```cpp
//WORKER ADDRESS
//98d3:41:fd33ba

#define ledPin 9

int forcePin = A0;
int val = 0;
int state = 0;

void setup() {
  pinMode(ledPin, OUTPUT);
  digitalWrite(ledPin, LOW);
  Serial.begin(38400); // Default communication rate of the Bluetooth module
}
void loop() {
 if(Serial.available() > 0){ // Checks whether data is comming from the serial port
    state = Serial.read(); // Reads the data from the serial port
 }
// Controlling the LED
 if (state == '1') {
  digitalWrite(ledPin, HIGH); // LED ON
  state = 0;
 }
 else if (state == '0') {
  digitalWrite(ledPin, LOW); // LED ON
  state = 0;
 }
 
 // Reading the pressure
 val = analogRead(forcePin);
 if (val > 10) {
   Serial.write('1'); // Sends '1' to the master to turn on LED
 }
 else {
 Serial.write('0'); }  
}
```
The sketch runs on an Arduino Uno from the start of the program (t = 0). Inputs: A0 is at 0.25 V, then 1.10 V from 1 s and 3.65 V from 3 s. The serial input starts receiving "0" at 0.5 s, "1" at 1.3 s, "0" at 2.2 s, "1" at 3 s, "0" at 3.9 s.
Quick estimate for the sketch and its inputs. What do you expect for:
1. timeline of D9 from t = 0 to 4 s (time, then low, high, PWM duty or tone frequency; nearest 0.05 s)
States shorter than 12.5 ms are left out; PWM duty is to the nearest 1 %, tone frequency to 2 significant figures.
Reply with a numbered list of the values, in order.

1. 0 s low; 1.3 s high; 2.2 s low; 3 s high; 3.9 s low
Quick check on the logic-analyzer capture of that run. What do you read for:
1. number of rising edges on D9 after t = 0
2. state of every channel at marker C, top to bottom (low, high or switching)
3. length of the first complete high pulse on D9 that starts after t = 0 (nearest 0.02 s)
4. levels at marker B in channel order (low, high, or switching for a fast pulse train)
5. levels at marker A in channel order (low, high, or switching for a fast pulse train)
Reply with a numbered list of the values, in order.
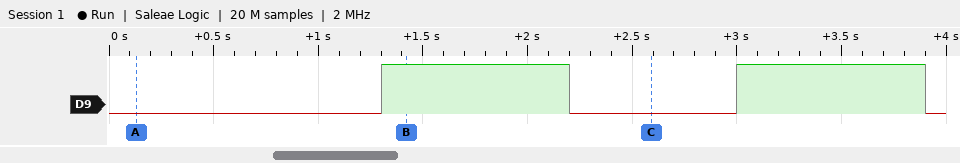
1. 2
2. D9 low
3. 0.90 s
4. D9 high
5. D9 low
